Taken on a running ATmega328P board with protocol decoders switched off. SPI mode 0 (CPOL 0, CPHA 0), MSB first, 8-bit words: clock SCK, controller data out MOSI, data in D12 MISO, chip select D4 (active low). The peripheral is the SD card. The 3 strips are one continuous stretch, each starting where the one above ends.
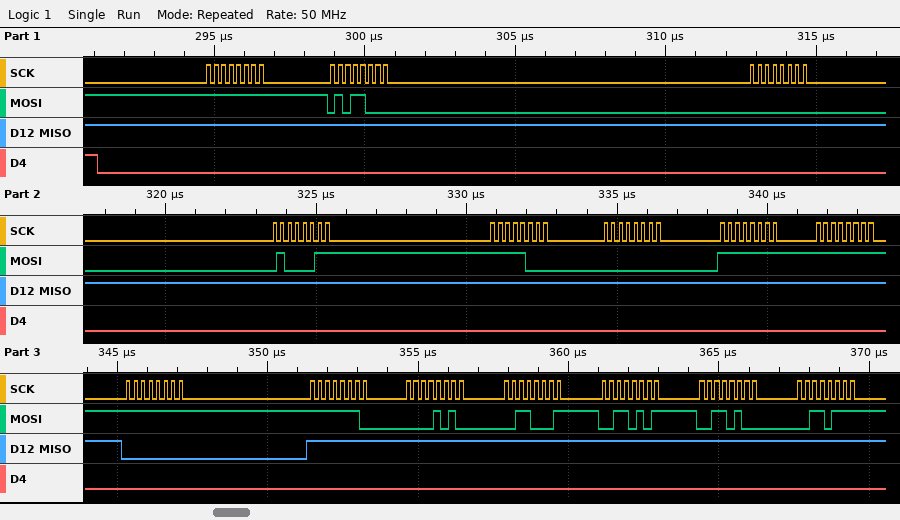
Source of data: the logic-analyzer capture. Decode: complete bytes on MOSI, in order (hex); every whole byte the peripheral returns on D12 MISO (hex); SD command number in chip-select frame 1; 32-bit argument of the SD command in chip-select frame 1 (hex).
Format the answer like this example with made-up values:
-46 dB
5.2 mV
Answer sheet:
FF 58 00 43 F8 00 FF FF FF FE 0A 31 35 34 37
FF FF FF FF FF FF FF FF 00 FF FF FF FF FF FF
CMD24
0x0043F800
